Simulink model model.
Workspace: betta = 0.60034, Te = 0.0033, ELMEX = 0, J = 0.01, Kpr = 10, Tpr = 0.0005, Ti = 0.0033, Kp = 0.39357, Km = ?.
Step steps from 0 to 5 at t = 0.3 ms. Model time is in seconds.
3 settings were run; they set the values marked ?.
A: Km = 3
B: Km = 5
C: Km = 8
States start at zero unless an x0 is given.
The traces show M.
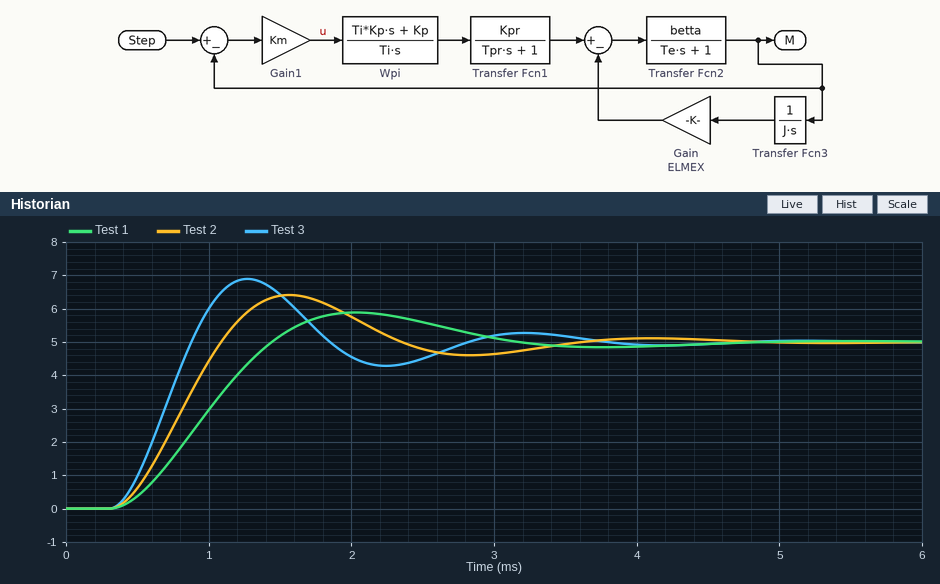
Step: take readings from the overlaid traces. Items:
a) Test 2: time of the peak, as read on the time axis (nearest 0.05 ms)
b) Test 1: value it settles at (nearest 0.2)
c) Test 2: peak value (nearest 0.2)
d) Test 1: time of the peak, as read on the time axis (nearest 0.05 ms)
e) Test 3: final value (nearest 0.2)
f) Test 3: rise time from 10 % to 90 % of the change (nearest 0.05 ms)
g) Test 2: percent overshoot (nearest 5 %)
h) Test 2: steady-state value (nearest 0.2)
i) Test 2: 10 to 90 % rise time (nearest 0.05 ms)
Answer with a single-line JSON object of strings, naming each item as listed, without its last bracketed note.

{"Test 2: time of the peak, as read on the time axis": "1.55 ms", "Test 1: value it settles at": "5.0", "Test 2: peak value": "6.4", "Test 1: time of the peak, as read on the time axis": "2.05 ms", "Test 3: final value": "5.0", "Test 3: rise time from 10 % to 90 % of the change": "0.40 ms", "Test 2: percent overshoot": "30 %", "Test 2: steady-state value": "5.0", "Test 2: 10 to 90 % rise time": "0.55 ms"}
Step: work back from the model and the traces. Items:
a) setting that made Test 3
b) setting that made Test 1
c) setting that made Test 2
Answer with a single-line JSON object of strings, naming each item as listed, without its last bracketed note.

{"setting that made Test 3": "C", "setting that made Test 1": "A", "setting that made Test 2": "B"}
